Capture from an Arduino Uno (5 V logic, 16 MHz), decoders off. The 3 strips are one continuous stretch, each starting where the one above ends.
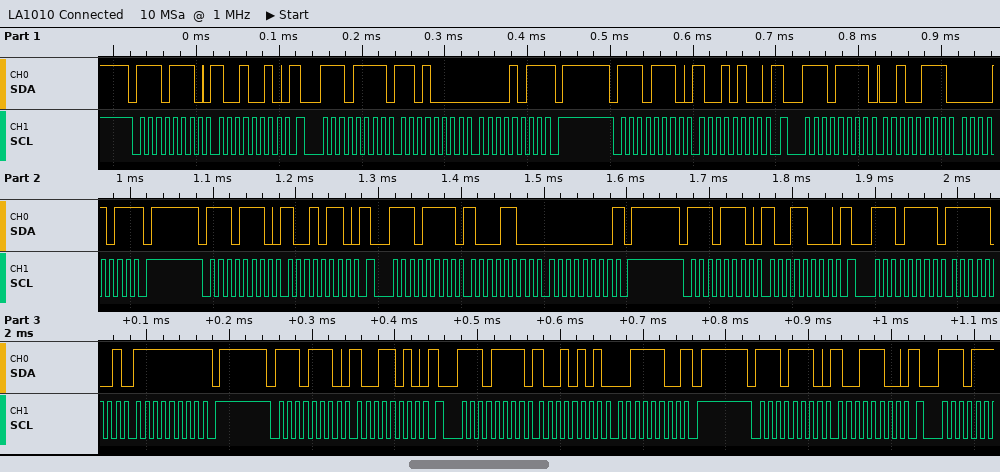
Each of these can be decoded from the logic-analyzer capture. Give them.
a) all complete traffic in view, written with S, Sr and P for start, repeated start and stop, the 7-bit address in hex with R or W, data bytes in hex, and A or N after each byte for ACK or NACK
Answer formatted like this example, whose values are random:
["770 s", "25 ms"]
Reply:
["S 77W A 92 A Sr 77R A D0 A 0B N P S 77W A 94 A Sr 77R A 27 A 0B N P S 77W A 96 A Sr 77R A 8C A 00 N P S 77W A 98 A Sr 77R A F9 A FF N P S 77W A 9A A Sr 77R A 95 A 3C N P S 77W A 9C A"]
